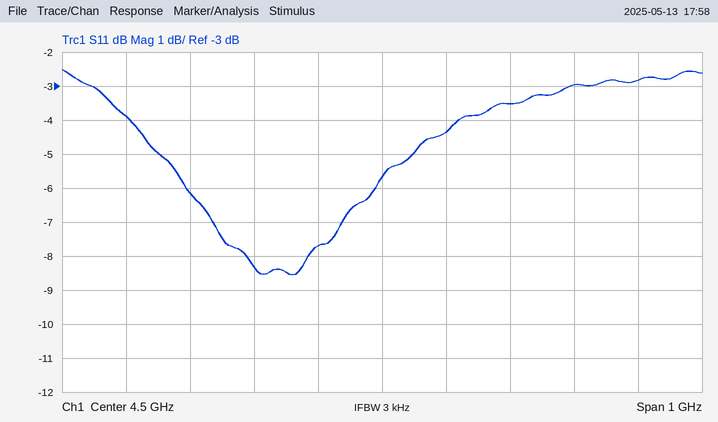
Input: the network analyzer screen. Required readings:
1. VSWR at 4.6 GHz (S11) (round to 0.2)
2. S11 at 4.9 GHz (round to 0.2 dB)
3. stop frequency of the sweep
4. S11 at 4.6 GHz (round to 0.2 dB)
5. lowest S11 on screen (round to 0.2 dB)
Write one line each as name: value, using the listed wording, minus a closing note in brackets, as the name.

VSWR at 4.6 GHz (S11): 4.0
S11 at 4.9 GHz: -2.8 dB
stop frequency of the sweep: 5 GHz
S11 at 4.6 GHz: -4.4 dB
lowest S11 on screen: -8.6 dB
